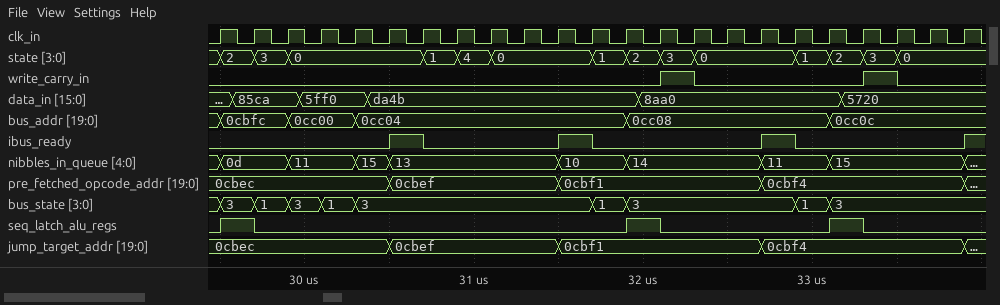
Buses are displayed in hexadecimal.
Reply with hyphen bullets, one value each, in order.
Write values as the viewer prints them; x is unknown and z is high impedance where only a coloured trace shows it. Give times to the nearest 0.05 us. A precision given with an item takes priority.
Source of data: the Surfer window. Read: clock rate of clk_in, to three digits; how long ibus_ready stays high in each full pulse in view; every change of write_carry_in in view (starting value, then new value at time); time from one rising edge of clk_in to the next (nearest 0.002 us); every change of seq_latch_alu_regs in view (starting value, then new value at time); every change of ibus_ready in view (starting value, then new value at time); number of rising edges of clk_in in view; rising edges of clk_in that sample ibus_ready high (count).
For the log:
- 5.00 MHz
- 0.2 us, 0.2 us, 0.2 us
- 0, 1 at 32.1 us, 0 at 32.3 us, 1 at 33.3 us, 0 at 33.5 us
- 0.2 us
- 0, 1 at 29.5 us, 0 at 29.7 us, 1 at 31.9 us, 0 at 32.1 us, 1 at 33.1 us, 0 at 33.3 us
- 0, 1 at 30.5 us, 0 at 30.7 us, 1 at 31.5 us, 0 at 31.7 us, 1 at 32.7 us, 0 at 32.9 us, 1 at 33.9 us
- 23
- 3
